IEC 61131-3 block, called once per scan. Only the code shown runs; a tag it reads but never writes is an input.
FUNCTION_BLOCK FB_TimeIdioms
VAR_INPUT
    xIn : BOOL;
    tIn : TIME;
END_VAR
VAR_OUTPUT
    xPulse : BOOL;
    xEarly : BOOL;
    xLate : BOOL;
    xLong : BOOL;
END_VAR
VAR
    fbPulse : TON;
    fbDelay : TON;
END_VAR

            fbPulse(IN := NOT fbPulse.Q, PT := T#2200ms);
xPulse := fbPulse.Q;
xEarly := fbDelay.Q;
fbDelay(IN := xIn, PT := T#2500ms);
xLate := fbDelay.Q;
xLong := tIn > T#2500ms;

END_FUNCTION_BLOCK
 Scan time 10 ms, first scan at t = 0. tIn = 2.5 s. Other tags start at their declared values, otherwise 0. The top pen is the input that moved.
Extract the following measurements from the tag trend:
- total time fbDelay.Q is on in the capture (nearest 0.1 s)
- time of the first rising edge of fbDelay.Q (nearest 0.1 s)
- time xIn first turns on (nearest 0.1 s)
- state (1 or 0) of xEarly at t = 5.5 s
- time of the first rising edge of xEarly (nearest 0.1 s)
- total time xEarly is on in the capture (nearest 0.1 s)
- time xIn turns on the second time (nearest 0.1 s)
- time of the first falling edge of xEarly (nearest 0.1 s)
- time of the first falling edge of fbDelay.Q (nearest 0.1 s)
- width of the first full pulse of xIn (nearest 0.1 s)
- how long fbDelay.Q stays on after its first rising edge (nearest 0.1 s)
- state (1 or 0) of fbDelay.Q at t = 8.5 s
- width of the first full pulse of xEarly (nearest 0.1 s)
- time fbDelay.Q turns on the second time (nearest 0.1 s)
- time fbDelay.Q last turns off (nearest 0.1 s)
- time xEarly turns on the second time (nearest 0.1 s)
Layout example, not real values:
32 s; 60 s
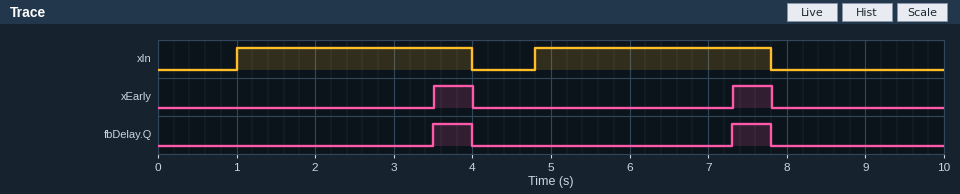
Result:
1.0 s; 3.5 s; 1.0 s; 0; 3.5 s; 1.0 s; 4.8 s; 4.0 s; 4.0 s; 3.0 s; 0.5 s; 0; 0.5 s; 7.3 s; 7.8 s; 7.3 s
